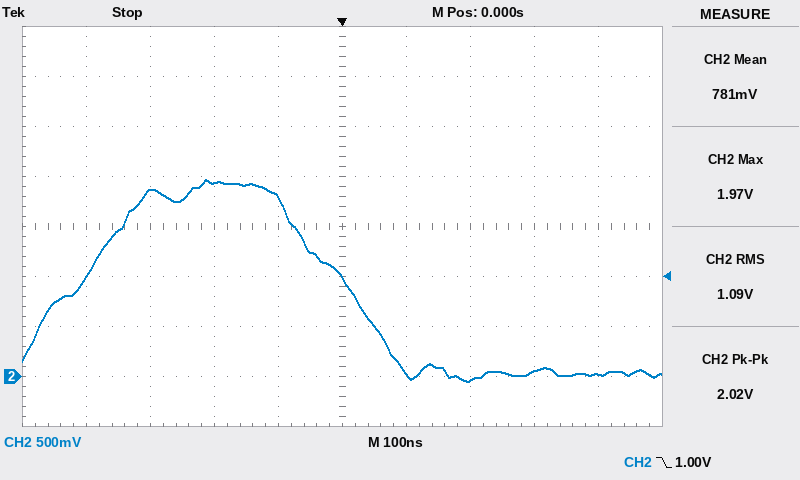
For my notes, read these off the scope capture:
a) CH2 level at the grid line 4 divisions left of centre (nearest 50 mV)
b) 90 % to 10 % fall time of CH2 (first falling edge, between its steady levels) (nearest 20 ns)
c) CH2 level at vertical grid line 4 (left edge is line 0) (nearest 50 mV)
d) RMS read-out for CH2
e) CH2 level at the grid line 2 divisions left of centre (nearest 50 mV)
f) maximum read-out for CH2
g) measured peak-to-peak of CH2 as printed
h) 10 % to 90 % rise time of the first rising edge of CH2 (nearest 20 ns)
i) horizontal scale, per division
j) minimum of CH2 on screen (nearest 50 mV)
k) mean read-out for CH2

1.00 V
180 ns
1.80 V
1.09 V
1.95 V
1.97 V
2.02 V
180 ns
100 ns
-50 mV
781 mV
